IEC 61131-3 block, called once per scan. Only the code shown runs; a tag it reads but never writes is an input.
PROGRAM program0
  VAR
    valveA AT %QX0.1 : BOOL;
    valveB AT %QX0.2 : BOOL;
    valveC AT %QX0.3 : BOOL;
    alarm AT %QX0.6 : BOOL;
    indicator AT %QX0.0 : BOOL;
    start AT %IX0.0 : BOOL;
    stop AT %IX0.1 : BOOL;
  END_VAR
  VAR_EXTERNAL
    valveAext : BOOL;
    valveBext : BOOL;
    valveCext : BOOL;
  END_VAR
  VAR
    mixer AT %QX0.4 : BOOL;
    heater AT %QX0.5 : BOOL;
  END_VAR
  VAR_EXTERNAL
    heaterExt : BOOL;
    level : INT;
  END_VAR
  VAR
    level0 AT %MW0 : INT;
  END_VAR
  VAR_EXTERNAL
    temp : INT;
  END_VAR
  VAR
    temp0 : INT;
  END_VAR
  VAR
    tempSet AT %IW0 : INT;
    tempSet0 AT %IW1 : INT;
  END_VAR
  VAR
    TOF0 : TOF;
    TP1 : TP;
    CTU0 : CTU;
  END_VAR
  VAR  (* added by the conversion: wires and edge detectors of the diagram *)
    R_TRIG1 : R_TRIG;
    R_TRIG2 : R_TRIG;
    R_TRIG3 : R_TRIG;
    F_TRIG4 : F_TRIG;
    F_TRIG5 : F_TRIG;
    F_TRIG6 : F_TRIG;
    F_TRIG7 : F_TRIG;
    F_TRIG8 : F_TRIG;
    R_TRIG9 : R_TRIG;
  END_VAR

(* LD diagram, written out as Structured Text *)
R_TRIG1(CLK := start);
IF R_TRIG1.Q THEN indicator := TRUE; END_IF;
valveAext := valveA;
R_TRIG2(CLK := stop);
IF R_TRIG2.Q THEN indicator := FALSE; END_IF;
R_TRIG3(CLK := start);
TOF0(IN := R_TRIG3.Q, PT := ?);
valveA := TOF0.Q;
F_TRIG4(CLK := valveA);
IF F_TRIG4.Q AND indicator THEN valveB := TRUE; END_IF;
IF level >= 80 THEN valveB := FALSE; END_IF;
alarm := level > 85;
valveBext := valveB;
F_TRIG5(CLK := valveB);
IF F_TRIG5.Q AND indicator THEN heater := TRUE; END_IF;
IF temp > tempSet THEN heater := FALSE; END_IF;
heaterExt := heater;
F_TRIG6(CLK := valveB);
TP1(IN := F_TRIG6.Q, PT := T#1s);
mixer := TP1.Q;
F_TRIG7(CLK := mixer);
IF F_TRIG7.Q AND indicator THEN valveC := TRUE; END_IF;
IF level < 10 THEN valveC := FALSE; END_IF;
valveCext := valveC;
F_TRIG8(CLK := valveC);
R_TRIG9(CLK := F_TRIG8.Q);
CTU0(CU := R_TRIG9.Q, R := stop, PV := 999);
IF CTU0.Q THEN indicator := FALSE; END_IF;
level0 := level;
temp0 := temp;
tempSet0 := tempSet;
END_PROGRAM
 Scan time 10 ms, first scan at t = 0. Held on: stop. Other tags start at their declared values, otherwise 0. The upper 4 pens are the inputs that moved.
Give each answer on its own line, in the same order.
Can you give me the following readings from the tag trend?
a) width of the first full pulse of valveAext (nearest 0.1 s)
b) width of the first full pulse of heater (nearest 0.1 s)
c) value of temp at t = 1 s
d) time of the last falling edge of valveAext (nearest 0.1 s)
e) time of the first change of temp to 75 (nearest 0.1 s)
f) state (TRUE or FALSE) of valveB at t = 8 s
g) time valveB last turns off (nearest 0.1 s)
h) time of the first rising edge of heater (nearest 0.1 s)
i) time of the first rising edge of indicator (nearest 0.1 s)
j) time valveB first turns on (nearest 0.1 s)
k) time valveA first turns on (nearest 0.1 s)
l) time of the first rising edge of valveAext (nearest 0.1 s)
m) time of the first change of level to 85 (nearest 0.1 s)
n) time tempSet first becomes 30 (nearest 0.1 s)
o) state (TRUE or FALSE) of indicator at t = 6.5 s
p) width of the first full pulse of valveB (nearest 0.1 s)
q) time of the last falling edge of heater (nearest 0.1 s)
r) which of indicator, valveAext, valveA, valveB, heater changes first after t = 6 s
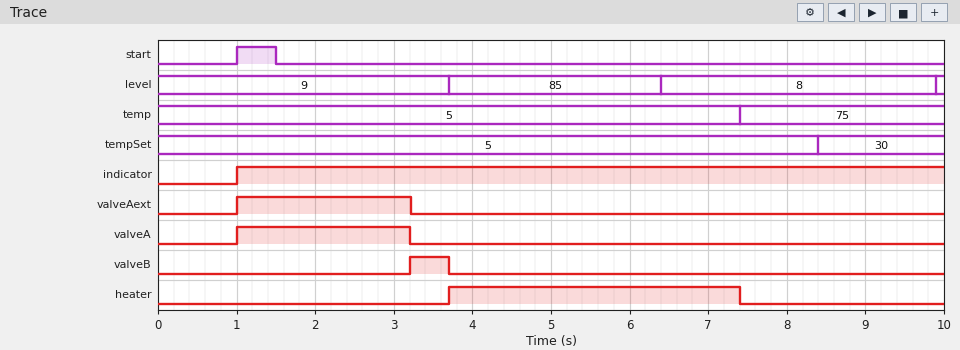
2.2 s
3.7 s
5
3.2 s
7.4 s
FALSE
3.7 s
3.7 s
1.0 s
3.2 s
1.0 s
1.0 s
3.7 s
8.4 s
TRUE
0.5 s
7.4 s
heater
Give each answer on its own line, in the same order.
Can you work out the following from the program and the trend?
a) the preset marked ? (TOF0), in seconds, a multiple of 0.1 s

2.2 s
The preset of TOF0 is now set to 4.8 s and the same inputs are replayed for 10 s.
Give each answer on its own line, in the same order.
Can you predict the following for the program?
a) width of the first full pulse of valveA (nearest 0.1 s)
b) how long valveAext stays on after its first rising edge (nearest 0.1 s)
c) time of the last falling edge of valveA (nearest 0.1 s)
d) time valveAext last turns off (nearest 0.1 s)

4.8 s
4.8 s
5.8 s
5.8 s
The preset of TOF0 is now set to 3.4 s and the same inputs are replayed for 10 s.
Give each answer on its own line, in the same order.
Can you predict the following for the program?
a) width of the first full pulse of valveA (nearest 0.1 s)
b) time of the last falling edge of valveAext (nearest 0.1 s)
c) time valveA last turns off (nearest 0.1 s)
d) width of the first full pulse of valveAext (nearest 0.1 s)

3.4 s
4.4 s
4.4 s
3.4 s
